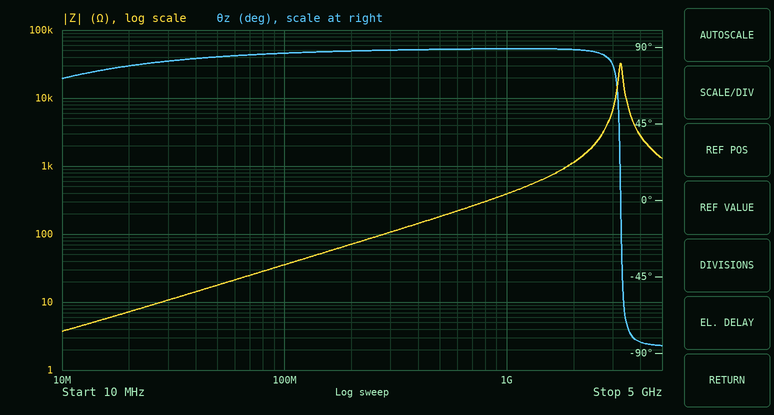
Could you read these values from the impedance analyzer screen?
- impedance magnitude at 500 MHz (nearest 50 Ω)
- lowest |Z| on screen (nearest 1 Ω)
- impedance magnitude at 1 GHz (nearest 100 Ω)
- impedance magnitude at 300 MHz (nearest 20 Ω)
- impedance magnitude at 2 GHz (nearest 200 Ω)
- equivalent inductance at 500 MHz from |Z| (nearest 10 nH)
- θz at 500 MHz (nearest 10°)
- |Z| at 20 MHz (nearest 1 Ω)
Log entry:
200 Ω
4 Ω
400 Ω
100 Ω
1.2 kΩ
60 nH
90°
7 Ω
